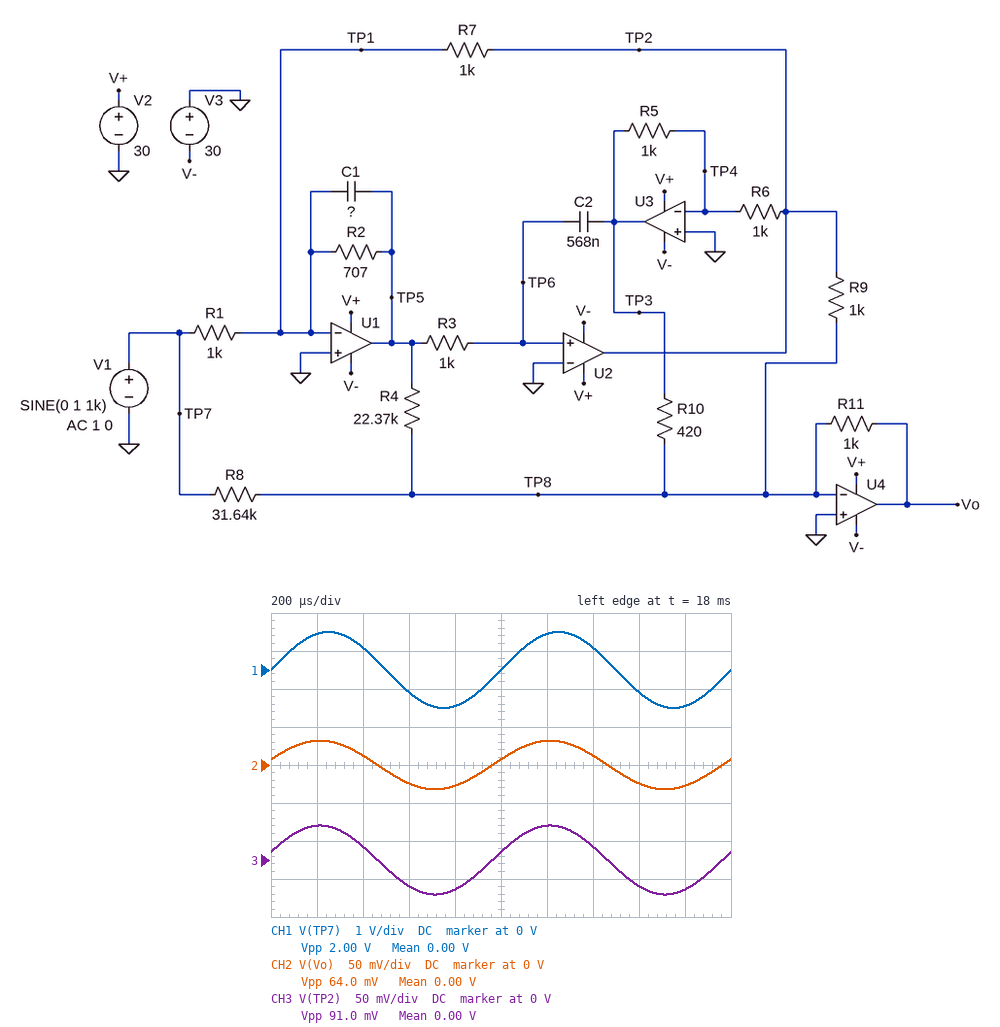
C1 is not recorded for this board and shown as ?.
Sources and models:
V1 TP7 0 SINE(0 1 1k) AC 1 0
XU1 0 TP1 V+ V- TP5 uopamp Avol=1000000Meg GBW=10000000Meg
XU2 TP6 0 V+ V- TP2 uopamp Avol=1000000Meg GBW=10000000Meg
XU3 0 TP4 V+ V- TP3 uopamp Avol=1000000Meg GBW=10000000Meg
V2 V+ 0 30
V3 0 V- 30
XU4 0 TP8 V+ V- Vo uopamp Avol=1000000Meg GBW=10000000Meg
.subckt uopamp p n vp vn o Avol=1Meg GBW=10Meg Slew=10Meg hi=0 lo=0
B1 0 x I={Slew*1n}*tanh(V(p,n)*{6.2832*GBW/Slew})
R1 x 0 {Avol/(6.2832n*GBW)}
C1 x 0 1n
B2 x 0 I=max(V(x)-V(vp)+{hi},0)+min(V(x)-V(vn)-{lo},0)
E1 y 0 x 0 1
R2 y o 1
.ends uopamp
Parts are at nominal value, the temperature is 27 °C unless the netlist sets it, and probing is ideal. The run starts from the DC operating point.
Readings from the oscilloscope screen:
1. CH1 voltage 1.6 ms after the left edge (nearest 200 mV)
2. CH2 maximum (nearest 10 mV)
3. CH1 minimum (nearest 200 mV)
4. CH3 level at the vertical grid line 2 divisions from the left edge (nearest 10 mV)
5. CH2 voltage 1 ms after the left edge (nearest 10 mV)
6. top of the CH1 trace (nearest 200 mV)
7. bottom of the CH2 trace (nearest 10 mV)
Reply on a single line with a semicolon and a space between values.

-600 mV; 30 mV; -1.0 V; 20 mV; 10 mV; 1.0 V; -30 mV
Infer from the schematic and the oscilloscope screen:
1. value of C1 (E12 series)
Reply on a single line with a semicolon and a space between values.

1 µF
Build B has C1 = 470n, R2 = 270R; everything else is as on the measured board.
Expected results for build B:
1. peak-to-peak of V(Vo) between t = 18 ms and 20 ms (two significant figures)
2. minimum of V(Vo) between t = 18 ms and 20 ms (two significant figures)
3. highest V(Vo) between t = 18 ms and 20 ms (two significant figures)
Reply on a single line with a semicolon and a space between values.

140 mV; -68 mV; 68 mV
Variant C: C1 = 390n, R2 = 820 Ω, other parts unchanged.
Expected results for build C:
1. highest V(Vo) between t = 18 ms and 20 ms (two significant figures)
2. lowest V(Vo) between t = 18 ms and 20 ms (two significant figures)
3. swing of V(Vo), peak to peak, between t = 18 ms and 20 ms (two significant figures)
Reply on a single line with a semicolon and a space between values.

130 mV; -130 mV; 260 mV
